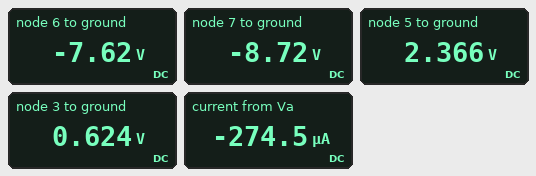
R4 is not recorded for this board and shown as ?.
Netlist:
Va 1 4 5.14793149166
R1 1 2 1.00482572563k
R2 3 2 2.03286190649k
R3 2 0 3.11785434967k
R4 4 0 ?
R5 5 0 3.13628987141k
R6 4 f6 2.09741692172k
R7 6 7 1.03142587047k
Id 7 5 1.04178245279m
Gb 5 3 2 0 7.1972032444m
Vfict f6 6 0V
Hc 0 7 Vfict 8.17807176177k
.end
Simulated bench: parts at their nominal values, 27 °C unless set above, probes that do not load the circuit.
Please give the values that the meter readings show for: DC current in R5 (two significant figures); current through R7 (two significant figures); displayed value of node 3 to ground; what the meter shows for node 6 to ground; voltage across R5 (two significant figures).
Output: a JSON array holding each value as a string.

["750 µA", "1.1 mA", "0.624 V", "-7.62 V", "2.4 V"]
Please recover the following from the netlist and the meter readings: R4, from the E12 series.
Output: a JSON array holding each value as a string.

["6.8 kΩ"]
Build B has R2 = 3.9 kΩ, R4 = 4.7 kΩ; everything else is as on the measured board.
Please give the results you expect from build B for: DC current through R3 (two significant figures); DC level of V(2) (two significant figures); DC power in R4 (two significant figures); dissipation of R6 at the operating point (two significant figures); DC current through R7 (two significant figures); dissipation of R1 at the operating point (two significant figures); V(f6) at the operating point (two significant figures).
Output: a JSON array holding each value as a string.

["3.5 µA", "-11 mV", "5.5 mW", "2.1 mW", "1.0 mA", "5.6 µW", "-7.2 V"]
